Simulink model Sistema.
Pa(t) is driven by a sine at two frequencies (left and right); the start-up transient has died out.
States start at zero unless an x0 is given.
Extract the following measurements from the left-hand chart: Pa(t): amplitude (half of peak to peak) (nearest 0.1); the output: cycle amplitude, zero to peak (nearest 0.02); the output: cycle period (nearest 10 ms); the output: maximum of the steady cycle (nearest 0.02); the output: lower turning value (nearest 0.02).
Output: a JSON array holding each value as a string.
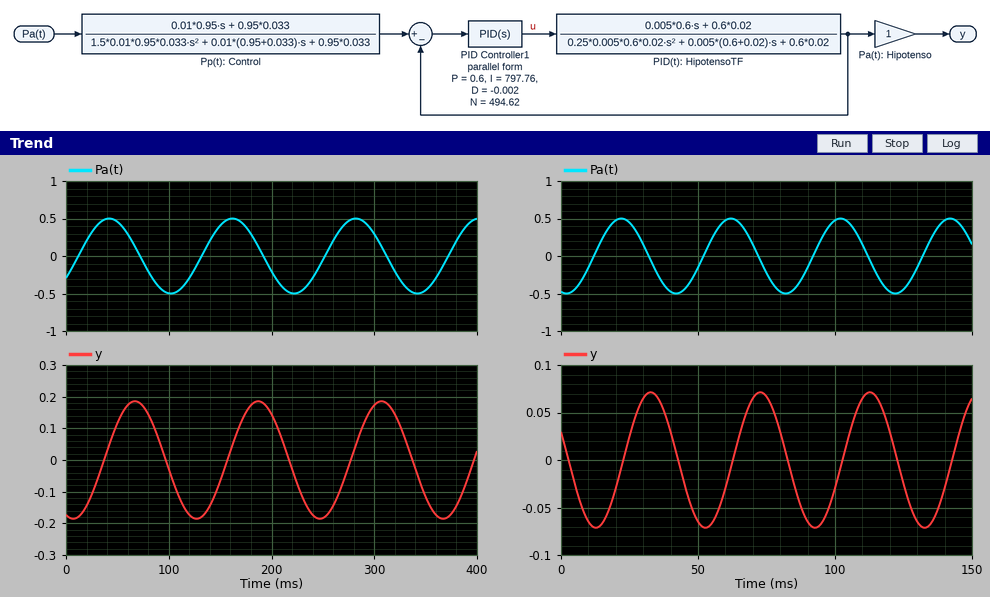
["0.5", "0.18", "120 ms", "0.18", "-0.18"]
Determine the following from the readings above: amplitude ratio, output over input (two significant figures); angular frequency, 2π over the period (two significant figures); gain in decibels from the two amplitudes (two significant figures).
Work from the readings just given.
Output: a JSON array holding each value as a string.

["0.36", "0.052 rad/ms", "-8.9 dB"]
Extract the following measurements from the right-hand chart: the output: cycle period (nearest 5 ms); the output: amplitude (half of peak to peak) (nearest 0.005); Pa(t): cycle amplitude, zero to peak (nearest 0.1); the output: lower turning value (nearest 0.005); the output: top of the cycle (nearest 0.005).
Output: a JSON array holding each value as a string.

["40 ms", "0.070", "0.5", "-0.070", "0.070"]
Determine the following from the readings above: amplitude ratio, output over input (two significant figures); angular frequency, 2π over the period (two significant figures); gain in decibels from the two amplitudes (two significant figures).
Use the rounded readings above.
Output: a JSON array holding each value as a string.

["0.14", "0.16 rad/ms", "-17 dB"]
